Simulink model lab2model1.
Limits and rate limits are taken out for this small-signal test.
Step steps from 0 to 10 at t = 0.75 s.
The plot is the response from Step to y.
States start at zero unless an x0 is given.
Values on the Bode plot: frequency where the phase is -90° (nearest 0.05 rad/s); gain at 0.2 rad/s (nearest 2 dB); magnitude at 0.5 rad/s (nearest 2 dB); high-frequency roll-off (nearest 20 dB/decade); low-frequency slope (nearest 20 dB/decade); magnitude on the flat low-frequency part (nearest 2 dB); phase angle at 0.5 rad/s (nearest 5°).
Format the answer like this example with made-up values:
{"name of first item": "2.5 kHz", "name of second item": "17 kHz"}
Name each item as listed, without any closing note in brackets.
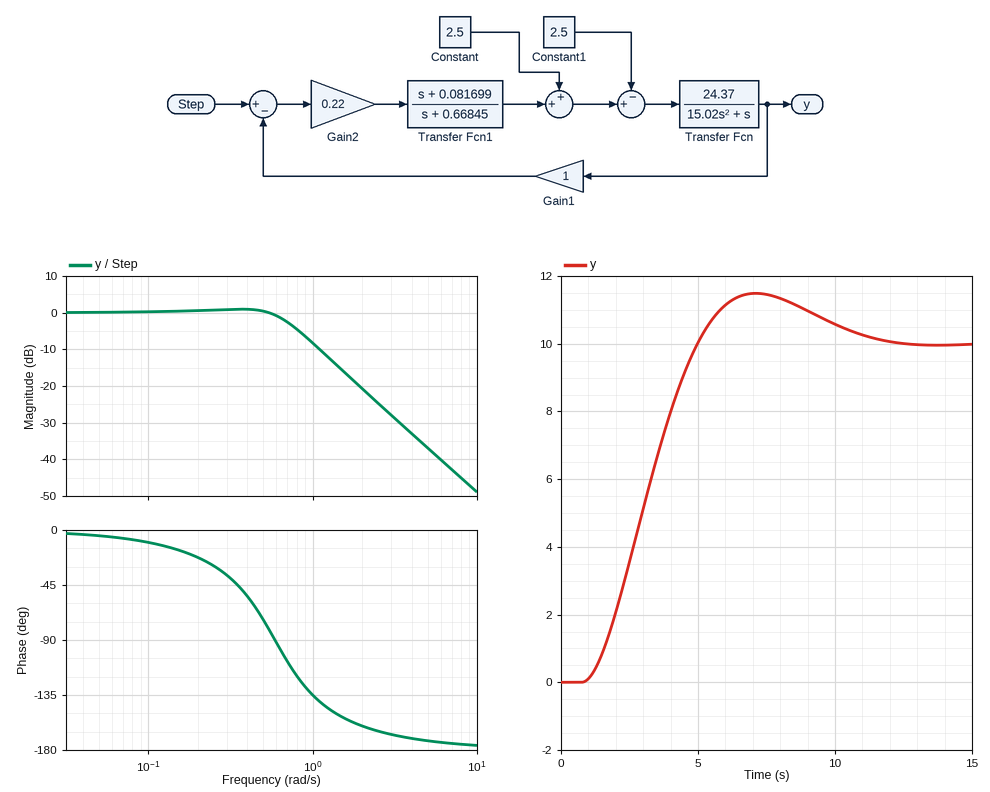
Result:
{"frequency where the phase is -90°": "0.60 rad/s", "gain at 0.2 rad/s": "0 dB", "magnitude at 0.5 rad/s": "0 dB", "high-frequency roll-off": "-40 dB/decade", "low-frequency slope": "0 dB/decade", "magnitude on the flat low-frequency part": "0 dB", "phase angle at 0.5 rad/s": "-75°"}
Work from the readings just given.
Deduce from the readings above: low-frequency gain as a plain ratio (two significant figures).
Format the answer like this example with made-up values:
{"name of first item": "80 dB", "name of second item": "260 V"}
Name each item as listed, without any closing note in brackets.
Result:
{"low-frequency gain as a plain ratio": "1.0"}
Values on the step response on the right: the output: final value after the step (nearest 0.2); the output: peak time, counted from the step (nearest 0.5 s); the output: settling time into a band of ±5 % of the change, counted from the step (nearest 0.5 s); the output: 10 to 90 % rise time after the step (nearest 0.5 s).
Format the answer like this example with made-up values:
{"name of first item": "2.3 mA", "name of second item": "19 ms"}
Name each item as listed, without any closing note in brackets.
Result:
{"the output: final value after the step": "10.0", "the output: peak time, counted from the step": "6.5 s", "the output: settling time into a band of ±5 % of the change, counted from the step": "9.5 s", "the output: 10 to 90 % rise time after the step": "3.0 s"}
